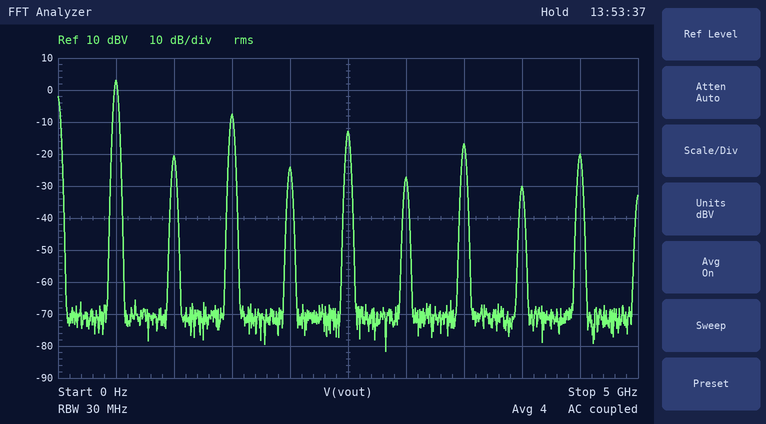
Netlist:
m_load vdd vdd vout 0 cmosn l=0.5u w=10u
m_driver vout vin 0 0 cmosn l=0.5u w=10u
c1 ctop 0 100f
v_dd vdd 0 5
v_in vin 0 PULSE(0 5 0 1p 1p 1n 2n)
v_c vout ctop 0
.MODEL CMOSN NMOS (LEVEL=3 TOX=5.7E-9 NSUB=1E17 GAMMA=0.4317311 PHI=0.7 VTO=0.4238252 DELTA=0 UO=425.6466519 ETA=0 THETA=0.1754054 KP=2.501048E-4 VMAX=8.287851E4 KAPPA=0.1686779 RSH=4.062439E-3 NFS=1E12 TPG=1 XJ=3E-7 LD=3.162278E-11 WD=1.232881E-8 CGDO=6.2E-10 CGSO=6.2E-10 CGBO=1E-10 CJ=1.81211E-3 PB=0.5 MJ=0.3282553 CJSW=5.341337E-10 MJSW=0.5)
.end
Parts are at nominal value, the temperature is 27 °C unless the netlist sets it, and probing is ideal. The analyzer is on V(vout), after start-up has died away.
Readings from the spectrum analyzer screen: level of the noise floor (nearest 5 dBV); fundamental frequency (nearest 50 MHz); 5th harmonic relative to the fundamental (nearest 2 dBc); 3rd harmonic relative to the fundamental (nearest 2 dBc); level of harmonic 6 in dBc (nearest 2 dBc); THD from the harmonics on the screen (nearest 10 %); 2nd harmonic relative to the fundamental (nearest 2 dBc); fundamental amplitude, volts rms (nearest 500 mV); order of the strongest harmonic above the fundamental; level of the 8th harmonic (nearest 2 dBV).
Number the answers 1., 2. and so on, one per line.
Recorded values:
1. -70 dBV
2. 500 MHz
3. -16 dBc
4. -10 dBc
5. -30 dBc
6. 40 %
7. -24 dBc
8. 1.5 V
9. 3
10. -30 dBV
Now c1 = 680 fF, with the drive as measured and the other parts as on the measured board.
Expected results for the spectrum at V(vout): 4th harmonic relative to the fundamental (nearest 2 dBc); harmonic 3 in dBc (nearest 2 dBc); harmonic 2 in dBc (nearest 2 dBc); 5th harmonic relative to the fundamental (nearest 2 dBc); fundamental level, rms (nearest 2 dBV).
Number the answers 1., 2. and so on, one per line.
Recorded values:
1. -36 dBc
2. -16 dBc
3. -22 dBc
4. -24 dBc
5. 0 dBV
